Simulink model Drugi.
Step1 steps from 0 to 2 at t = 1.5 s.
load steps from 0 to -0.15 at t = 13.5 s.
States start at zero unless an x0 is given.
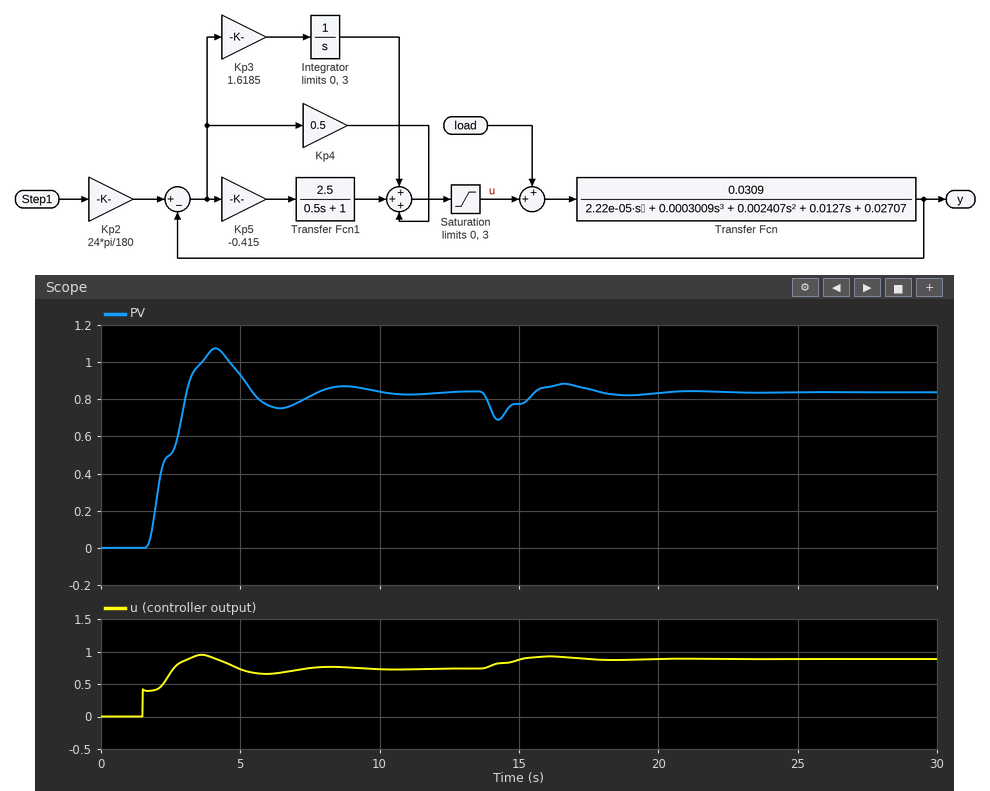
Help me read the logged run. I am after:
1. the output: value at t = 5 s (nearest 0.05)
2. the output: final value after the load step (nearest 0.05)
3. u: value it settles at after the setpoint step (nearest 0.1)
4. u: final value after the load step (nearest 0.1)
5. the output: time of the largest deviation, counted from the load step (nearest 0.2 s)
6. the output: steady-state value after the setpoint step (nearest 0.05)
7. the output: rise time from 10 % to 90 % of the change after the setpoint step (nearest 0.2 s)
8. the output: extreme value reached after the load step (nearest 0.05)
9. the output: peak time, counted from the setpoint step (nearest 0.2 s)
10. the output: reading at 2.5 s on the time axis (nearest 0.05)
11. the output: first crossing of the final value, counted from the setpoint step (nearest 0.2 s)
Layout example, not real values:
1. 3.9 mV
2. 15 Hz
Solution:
1. 0.95
2. 0.85
3. 0.7
4. 0.9
5. 0.8 s
6. 0.85
7. 1.2 s
8. 0.70
9. 2.6 s
10. 0.50
11. 1.6 s
